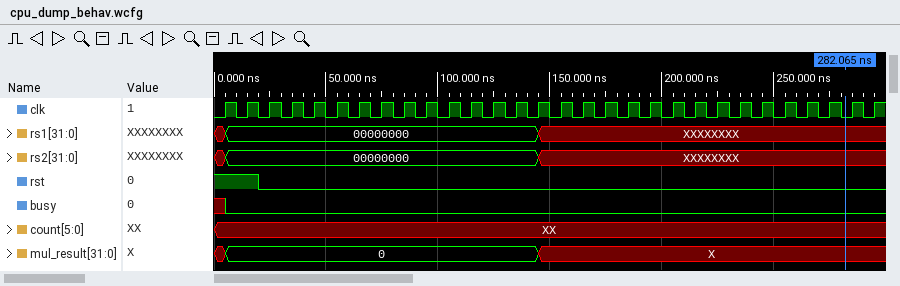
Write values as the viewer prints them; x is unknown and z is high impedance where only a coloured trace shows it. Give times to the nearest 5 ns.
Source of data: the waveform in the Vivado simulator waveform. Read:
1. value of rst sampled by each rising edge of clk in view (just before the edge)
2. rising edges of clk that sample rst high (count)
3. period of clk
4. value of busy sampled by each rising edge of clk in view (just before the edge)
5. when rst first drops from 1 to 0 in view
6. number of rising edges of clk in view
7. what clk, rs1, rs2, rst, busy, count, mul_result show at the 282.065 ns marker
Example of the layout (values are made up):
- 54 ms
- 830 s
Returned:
- 1 1 0 0 0 0 0 0 0 0 0 0 0 0 0 0 0 0 0 0 0 0 0 0 0 0 0 0 0 0
- 2
- 10 ns
- x 0 0 0 0 0 0 0 0 0 0 0 0 0 0 0 0 0 0 0 0 0 0 0 0 0 0 0 0 0
- 20 ns
- 30
- clk=0, rs1=XXXXXXXX, rs2=XXXXXXXX, rst=0, busy=0, count=XX, mul_result=X
